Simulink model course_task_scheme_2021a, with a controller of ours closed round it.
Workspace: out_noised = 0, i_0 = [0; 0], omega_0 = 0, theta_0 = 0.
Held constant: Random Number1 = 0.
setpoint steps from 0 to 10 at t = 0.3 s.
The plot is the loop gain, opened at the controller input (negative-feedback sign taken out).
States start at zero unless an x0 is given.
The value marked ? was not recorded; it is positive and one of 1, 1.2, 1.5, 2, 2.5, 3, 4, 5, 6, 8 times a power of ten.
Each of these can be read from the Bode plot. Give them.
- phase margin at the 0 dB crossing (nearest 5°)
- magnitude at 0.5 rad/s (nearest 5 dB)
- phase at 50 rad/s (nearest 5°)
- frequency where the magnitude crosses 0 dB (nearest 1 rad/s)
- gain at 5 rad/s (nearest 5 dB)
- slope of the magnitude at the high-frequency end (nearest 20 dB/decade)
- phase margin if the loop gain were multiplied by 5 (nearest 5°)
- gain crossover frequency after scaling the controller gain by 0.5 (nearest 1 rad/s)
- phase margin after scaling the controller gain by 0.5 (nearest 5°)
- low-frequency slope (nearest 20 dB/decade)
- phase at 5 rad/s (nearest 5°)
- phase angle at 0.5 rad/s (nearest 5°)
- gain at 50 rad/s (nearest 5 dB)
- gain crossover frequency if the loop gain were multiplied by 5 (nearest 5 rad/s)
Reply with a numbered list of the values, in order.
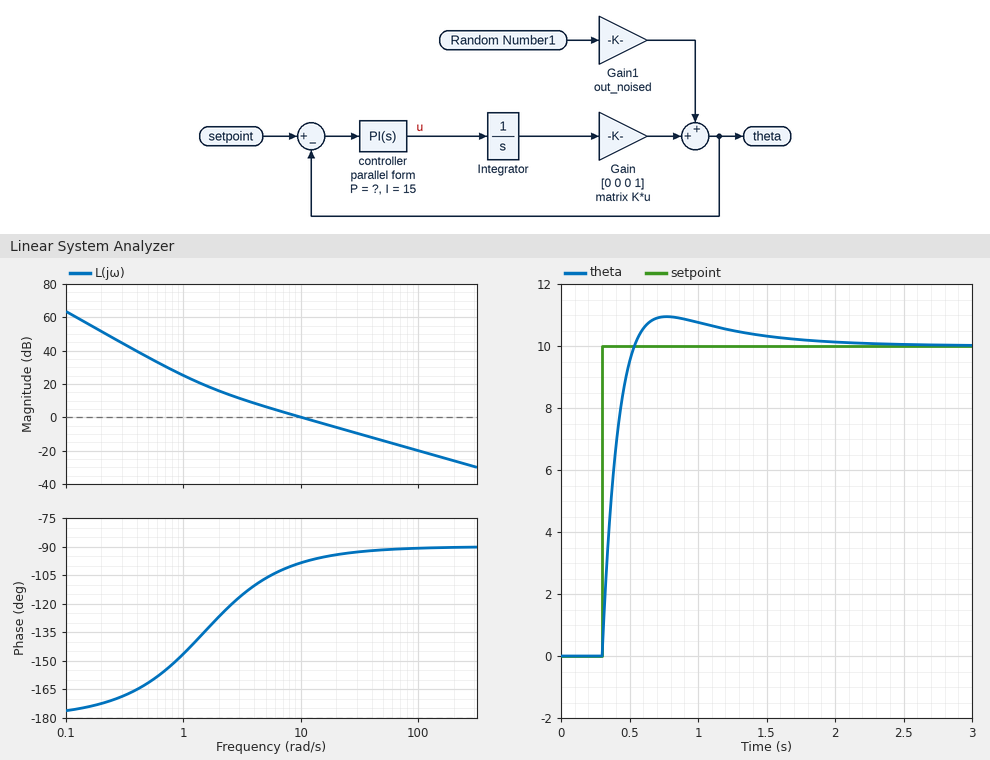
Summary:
1. 80°
2. 35 dB
3. -90°
4. 10 rad/s
5. 5 dB
6. -20 dB/decade
7. 90°
8. 5 rad/s
9. 75°
10. -40 dB/decade
11. -105°
12. -160°
13. -15 dB
14. 50 rad/s
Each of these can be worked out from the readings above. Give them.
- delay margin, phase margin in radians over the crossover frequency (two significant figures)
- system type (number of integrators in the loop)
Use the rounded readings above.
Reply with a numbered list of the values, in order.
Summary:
1. 0.14 s
2. 2
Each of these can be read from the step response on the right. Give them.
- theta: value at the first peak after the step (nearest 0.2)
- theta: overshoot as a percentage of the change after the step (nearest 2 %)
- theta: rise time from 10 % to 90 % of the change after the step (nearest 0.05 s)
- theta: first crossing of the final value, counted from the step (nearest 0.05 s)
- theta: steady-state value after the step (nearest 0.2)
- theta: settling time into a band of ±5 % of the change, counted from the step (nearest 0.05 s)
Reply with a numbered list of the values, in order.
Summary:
1. 11.0
2. 10 %
3. 0.15 s
4. 0.25 s
5. 10.0
6. 0.95 s
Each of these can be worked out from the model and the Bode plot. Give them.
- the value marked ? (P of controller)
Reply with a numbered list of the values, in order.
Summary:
1. 10
